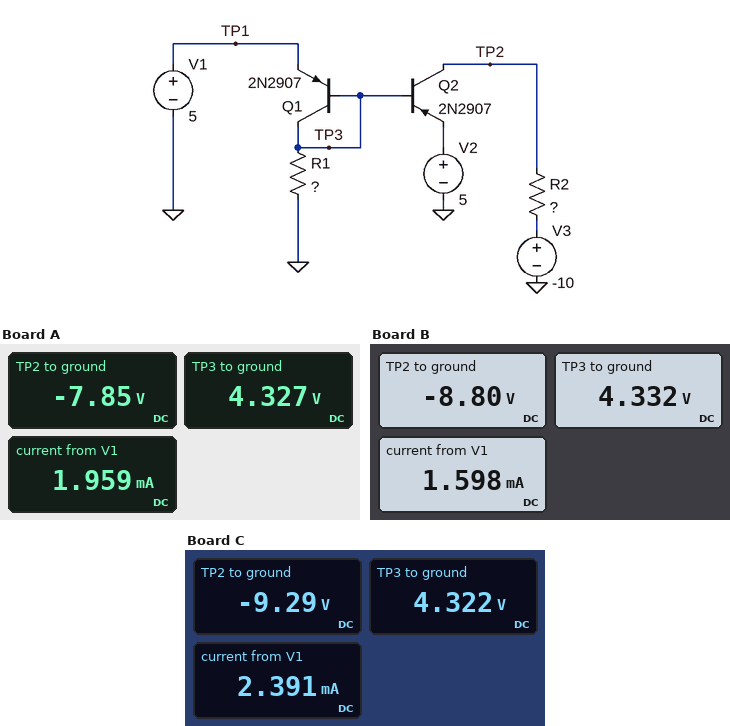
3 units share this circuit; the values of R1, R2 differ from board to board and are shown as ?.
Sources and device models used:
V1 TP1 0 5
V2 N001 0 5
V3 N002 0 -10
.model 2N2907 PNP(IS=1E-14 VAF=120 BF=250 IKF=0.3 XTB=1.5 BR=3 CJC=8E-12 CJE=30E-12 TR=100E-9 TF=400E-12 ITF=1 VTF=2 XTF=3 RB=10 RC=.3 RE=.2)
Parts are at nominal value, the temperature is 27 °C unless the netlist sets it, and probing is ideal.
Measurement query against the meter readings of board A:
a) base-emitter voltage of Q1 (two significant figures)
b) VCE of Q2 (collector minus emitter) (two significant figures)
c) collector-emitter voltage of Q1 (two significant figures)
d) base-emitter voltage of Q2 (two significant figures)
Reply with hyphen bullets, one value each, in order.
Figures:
- -670 mV
- -13 V
- -670 mV
- -670 mV
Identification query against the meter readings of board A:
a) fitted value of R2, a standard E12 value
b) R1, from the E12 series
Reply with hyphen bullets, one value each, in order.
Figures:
- 1 kΩ
- 2.2 kΩ
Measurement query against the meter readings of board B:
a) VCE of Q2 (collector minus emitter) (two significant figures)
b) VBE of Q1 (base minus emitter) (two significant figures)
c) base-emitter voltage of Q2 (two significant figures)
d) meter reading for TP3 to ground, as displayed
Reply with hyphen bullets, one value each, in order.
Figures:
- -14 V
- -670 mV
- -670 mV
- 4.332 V
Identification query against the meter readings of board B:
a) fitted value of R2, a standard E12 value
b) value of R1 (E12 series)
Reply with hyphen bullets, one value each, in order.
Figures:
- 680 Ω
- 2.7 kΩ
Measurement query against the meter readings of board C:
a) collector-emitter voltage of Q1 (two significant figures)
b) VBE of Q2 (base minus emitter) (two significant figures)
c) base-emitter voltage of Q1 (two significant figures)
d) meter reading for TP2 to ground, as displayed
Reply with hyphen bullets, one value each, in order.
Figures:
- -680 mV
- -680 mV
- -680 mV
- -9.29 V
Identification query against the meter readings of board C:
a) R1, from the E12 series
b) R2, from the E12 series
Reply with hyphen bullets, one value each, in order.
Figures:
- 1.8 kΩ
- 270 Ω
